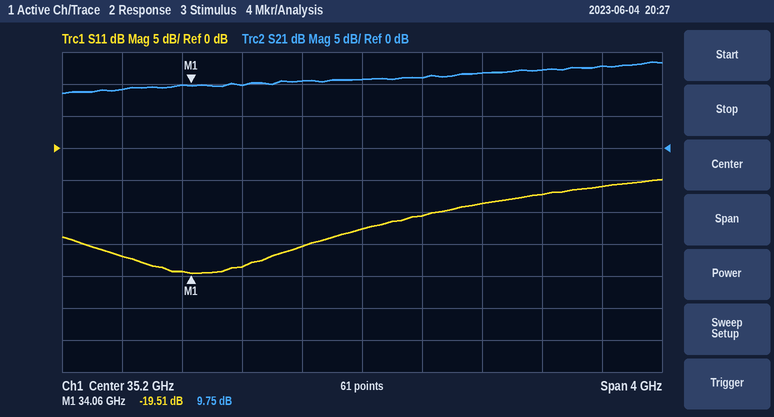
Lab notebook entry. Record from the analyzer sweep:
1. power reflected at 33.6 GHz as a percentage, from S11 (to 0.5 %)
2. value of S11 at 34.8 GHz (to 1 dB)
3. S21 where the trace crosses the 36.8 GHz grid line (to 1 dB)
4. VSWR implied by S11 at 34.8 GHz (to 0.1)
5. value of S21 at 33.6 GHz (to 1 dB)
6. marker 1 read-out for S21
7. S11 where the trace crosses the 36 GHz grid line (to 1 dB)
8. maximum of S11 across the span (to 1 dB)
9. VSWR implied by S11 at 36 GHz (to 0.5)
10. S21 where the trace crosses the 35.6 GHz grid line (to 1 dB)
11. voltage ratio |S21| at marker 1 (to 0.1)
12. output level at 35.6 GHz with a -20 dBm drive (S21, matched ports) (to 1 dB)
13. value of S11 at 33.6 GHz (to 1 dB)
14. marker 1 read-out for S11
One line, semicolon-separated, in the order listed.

2.0 %; -15 dB; 13 dB; 1.4; 9 dB; 9.75 dB; -9 dB; -5 dB; 2.0; 11 dB; 3.1; -9 dBm; -17 dB; -19.51 dB
